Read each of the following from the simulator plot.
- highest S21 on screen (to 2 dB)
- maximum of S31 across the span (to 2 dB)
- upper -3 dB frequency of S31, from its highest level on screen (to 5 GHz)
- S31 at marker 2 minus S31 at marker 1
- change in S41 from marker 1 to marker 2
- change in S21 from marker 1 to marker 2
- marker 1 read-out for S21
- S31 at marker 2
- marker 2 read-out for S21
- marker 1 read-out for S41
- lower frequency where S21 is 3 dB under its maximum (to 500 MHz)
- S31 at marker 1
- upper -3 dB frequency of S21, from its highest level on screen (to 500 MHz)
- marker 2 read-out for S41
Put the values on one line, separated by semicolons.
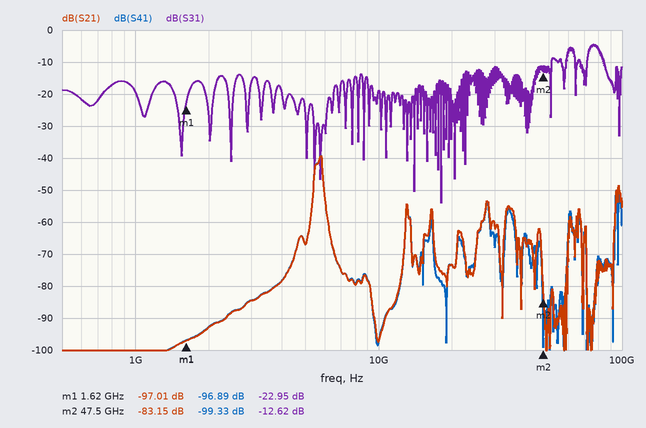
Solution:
-40 dB; -4 dB; 80 GHz; 10.33 dB; -2.44 dB; 13.86 dB; -97.01 dB; -12.62 dB; -83.15 dB; -96.89 dB; 5.5 GHz; -22.95 dB; 6.0 GHz; -99.33 dB
